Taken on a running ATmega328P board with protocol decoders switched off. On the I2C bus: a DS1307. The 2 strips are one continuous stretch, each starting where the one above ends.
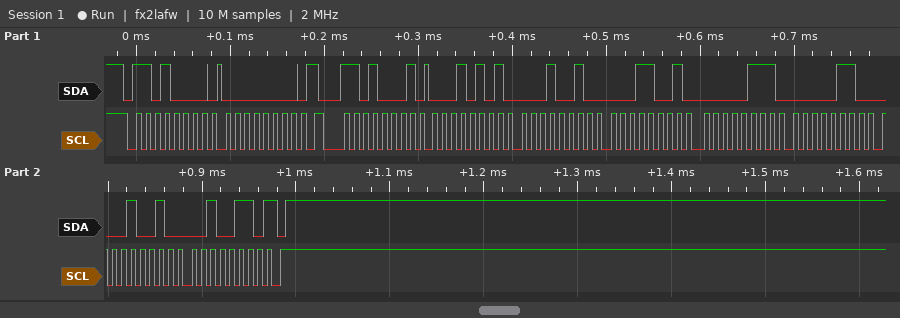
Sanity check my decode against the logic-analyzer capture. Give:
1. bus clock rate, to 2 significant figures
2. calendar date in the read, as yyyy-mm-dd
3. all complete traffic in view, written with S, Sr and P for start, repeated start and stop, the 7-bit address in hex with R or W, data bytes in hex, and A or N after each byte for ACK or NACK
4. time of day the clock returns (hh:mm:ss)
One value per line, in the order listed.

100 kHz
2026-12-06
S 68W A 00 A Sr 68R A 15 A 12 A 19 A 07 A 06 A 12 A 26 N P
19:12:15
